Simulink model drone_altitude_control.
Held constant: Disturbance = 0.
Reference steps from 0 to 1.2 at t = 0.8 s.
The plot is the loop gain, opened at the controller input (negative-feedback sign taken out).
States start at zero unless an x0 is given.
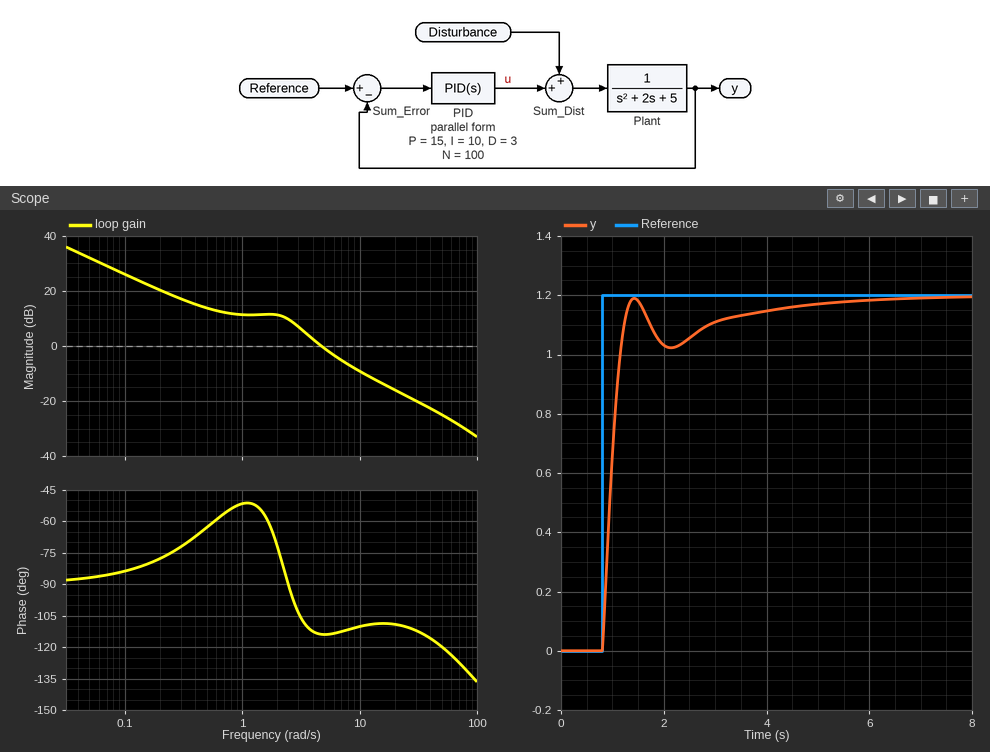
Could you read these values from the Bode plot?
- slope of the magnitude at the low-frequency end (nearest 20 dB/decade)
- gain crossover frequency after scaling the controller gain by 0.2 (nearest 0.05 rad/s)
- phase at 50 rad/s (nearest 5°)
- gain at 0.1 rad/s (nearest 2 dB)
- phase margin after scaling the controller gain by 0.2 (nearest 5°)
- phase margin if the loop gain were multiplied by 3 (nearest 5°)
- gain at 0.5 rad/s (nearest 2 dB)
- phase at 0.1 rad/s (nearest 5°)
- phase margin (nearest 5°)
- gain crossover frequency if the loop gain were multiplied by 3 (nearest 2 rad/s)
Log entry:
-20 dB/decade
0.50 rad/s
-120°
26 dB
115°
70°
14 dB
-85°
65°
10 rad/s
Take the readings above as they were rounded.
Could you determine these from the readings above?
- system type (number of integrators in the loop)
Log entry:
1
